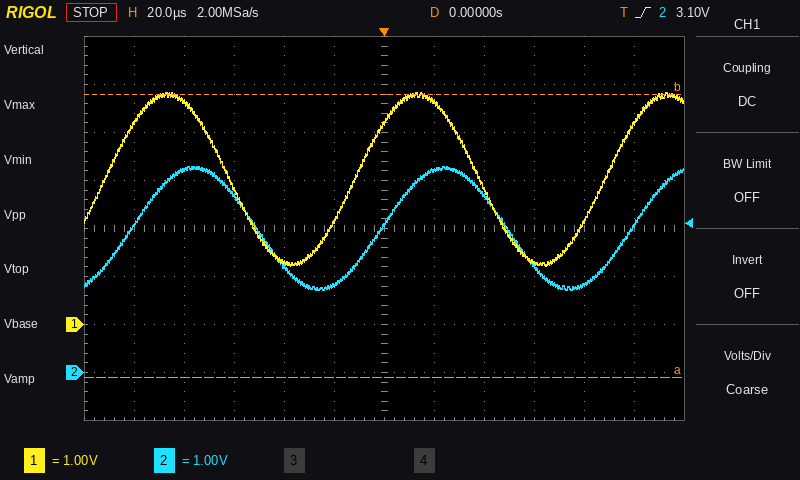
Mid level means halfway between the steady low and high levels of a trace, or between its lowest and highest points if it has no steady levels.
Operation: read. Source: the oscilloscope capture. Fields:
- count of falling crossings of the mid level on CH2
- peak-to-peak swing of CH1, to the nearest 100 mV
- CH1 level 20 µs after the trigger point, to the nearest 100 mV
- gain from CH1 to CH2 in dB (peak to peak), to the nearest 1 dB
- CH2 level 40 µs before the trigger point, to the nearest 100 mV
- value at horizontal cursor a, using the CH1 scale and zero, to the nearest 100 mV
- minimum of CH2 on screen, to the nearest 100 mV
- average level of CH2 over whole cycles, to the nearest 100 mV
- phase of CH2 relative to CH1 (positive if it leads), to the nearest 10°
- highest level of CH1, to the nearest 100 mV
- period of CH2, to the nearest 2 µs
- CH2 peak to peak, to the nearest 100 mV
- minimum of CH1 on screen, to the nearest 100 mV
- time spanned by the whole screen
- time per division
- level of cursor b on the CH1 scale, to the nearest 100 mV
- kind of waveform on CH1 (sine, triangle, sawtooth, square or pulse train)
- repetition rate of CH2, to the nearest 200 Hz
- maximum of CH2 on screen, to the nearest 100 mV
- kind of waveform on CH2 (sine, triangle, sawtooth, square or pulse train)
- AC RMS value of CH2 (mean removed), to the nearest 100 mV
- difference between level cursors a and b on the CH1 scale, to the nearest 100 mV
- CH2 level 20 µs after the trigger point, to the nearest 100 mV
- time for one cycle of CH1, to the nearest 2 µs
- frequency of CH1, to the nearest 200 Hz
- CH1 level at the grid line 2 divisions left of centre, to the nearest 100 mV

2
3.6 V
4.6 V
-3 dB
2.2 V
-1.1 V
1.7 V
3.0 V
-40°
4.8 V
100 µs
2.6 V
1.2 V
240 µs
20 µs
4.8 V
sine
10.0 kHz
4.3 V
sine
900 mV
5.9 V
4.2 V
100 µs
10.0 kHz
1.3 V
